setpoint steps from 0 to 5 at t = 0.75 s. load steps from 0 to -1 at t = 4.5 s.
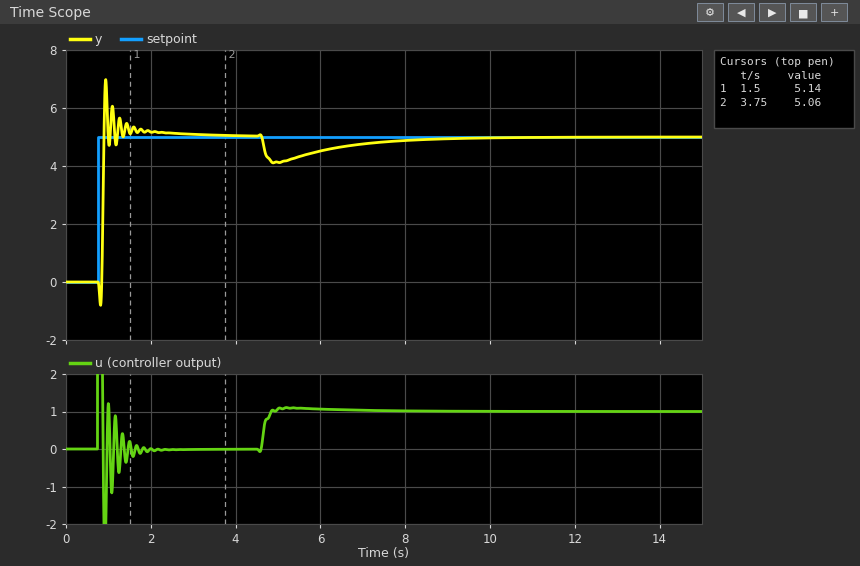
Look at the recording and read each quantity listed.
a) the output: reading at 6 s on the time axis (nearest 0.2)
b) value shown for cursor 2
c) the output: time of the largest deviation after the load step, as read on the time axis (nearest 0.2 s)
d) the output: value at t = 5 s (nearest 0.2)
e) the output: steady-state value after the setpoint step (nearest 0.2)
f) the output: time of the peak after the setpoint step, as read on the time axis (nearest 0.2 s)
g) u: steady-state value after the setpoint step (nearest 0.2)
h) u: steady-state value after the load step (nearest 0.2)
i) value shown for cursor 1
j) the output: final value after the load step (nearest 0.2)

4.6
5.06
4.8 s
4.2
5.0
1.0 s
0.0
1.0
5.14
5.0
